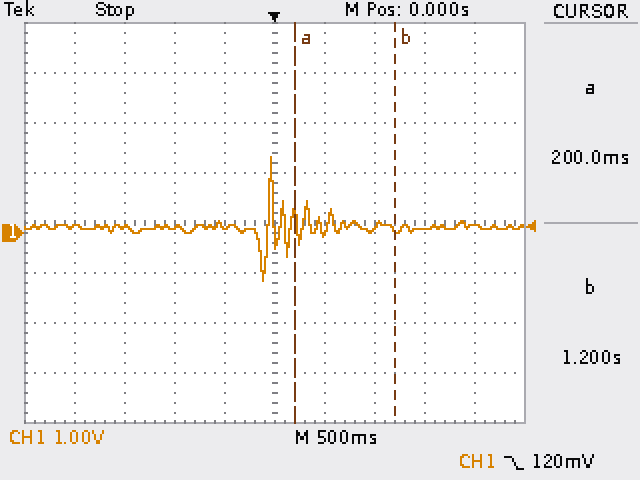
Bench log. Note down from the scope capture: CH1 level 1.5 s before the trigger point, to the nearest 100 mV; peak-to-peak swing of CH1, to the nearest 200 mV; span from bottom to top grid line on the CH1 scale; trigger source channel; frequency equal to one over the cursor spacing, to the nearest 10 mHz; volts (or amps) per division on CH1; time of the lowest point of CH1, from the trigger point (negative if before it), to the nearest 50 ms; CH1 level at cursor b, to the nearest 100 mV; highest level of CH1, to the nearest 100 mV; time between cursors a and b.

100 mV
2.4 V
8 V
CH1
1.00 Hz
1 V
-100 ms
100 mV
1.5 V
1.00 s
